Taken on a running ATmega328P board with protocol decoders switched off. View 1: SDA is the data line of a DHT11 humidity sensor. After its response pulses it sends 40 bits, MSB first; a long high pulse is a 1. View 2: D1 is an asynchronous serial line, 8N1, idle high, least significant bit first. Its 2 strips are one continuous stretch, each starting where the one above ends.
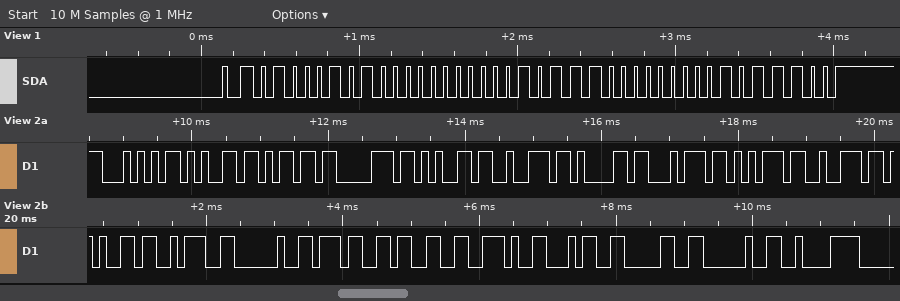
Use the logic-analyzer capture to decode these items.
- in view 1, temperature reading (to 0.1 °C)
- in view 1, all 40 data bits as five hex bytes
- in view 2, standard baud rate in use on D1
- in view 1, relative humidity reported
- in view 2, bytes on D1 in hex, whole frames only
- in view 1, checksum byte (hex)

23.0 °C
45 00 17 00 5C
9600 baud
69 %
0x54 0x65 0x6D 0x70 0x65 0x72 0x61 0x74 0x75 0x72 0x65 0x3A 0x20 0x37 0x33 0x2E 0x34 0x30 0x20 0xC2
0x5C
